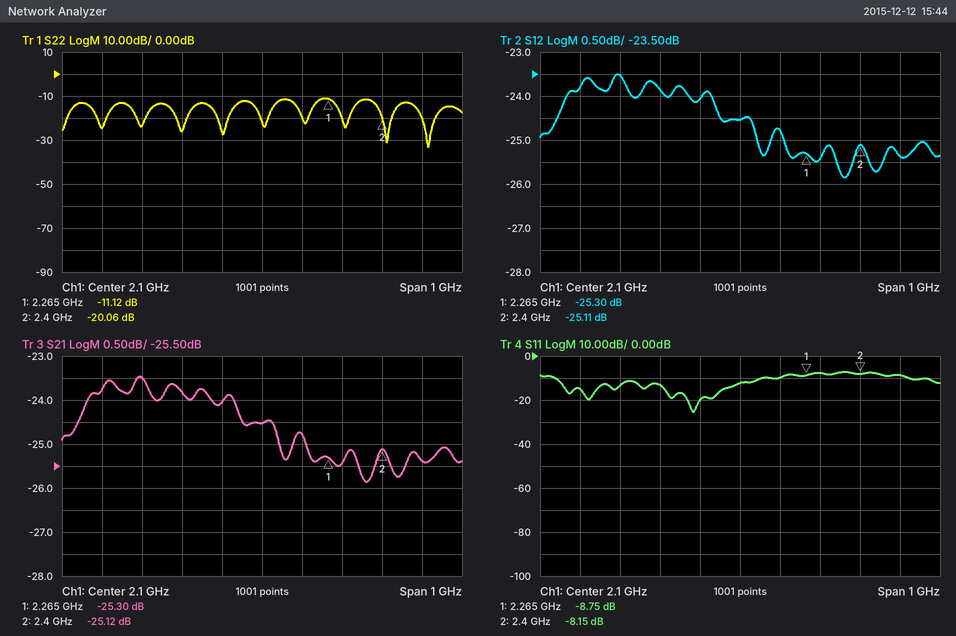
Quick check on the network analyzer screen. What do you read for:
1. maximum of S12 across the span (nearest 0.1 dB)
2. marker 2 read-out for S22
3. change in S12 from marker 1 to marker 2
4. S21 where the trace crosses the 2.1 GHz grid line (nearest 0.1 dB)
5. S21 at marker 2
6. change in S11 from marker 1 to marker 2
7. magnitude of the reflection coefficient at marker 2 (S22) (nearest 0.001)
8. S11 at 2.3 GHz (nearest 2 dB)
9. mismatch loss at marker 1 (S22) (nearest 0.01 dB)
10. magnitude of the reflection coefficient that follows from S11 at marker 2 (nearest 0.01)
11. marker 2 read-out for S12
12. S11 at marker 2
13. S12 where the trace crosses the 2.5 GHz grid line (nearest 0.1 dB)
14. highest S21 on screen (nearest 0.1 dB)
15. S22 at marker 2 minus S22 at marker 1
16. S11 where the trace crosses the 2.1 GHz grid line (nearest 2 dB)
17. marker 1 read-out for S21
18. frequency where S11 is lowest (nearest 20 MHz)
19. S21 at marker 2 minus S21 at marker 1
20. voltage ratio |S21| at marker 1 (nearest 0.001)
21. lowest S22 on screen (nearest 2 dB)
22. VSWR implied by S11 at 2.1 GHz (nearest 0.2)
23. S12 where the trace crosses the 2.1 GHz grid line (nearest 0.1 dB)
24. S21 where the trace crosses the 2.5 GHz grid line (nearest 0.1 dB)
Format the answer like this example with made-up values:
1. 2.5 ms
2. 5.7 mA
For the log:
1. -23.5 dB
2. -20.06 dB
3. 0.19 dB
4. -24.5 dB
5. -25.12 dB
6. 0.60 dB
7. 0.099
8. -8 dB
9. 0.35 dB
10. 0.39
11. -25.11 dB
12. -8.15 dB
13. -25.4 dB
14. -23.5 dB
15. -8.94 dB
16. -12 dB
17. -25.30 dB
18. 1.98 GHz
19. 0.18 dB
20. 0.054
21. -34 dB
22. 1.6
23. -24.5 dB
24. -25.4 dB
